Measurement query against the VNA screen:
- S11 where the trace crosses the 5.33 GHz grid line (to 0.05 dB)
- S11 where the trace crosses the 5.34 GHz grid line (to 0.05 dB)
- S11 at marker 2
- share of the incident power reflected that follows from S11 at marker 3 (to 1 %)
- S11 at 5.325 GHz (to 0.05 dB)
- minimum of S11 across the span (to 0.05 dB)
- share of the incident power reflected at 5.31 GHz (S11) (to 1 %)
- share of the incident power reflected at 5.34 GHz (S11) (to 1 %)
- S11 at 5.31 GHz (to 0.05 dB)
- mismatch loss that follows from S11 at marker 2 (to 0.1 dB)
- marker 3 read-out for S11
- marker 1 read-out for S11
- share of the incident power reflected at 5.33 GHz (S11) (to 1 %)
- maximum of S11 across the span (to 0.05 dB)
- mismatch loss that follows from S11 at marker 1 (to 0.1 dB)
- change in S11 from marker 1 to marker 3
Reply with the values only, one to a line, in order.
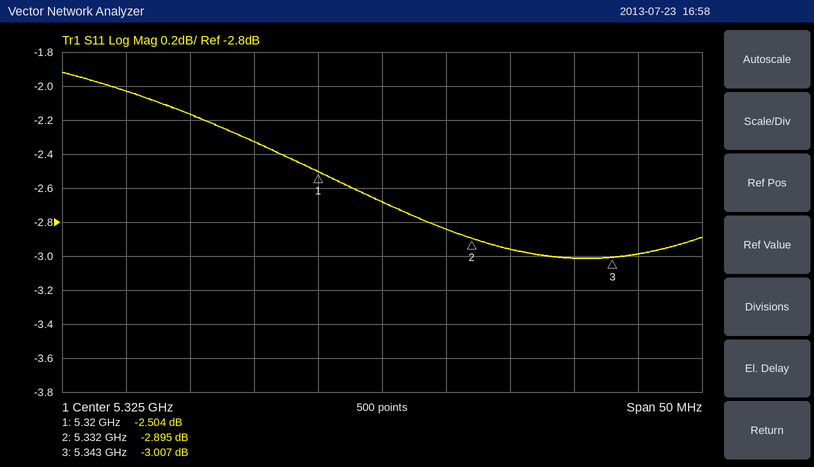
-2.85 dB
-3.00 dB
-2.895 dB
50 %
-2.70 dB
-3.00 dB
61 %
50 %
-2.15 dB
3.1 dB
-3.007 dB
-2.504 dB
52 %
-1.90 dB
3.6 dB
-0.503 dB
